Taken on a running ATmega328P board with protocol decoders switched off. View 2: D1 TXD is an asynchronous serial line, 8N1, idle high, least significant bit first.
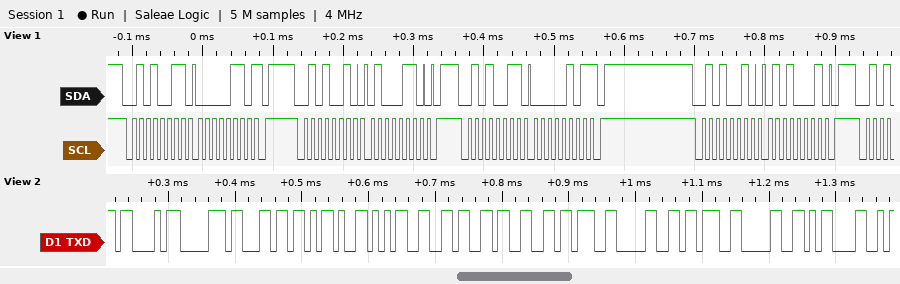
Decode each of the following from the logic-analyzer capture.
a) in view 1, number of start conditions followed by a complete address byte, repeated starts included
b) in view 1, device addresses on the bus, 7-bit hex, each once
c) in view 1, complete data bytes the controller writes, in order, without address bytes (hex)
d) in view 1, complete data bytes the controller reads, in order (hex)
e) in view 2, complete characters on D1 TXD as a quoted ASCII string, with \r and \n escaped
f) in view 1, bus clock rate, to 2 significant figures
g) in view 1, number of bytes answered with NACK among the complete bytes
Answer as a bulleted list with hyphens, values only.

- 4
- 0x29
- 46 51
- 06 05
- "Cpl-563;0;0\r"
- 100 kHz
- 2
